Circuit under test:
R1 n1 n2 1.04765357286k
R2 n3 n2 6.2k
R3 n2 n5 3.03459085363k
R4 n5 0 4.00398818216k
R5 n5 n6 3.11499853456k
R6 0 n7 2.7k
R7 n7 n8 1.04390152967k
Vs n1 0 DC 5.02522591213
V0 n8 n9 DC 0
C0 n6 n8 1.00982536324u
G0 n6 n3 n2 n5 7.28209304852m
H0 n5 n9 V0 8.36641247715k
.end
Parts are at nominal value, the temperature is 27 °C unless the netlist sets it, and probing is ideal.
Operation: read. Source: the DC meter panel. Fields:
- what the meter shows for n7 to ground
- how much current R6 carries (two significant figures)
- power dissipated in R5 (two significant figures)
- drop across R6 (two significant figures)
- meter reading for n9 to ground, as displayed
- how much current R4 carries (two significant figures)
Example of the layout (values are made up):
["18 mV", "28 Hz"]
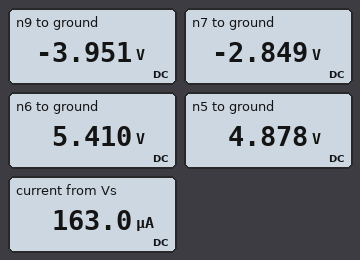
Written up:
["-2.849 V", "1.1 mA", "91 µW", "2.8 V", "-3.951 V", "1.2 mA"]
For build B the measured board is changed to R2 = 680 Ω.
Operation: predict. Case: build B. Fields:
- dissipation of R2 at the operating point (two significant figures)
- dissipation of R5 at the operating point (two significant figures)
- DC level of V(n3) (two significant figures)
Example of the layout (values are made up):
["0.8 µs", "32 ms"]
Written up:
["20 µW", "91 µW", "4.7 V"]
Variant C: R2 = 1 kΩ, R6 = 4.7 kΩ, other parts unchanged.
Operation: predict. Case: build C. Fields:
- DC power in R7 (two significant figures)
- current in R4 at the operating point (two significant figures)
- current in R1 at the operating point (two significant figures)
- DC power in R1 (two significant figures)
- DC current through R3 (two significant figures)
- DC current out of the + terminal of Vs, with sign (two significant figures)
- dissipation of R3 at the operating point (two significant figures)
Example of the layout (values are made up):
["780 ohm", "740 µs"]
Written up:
["4.9 mW", "1.4 mA", "750 µA", "590 µW", "36 µA", "-750 µA", "3.8 µW"]
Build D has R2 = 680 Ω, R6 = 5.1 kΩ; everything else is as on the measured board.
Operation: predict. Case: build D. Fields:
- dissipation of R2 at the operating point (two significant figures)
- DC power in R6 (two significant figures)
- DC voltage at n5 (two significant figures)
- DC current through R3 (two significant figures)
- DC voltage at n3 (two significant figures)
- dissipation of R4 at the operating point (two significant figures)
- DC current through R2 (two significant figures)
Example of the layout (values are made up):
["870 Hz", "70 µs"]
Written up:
["1.1 mW", "39 mW", "6.1 V", "58 µA", "7.2 V", "9.4 mW", "1.3 mA"]
